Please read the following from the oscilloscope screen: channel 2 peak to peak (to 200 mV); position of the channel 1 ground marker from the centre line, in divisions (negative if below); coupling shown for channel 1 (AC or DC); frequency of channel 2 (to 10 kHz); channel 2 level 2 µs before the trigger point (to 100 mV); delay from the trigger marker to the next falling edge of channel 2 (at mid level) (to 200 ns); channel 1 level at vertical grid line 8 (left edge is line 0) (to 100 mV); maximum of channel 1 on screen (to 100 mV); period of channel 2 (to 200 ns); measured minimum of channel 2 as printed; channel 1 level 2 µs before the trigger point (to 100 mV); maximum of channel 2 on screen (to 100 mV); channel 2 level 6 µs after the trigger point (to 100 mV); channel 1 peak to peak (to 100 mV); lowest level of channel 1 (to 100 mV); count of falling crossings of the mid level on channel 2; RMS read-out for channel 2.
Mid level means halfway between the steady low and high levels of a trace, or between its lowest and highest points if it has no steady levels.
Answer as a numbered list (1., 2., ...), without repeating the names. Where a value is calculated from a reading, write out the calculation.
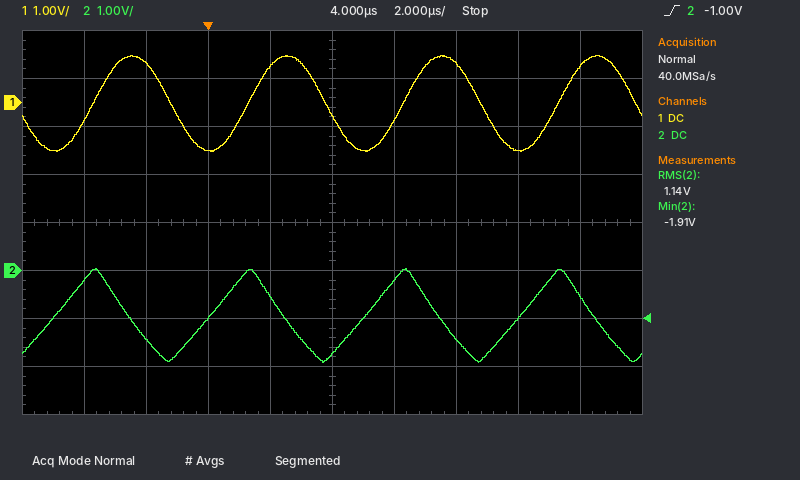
1. 2.0 V
2. +2.5 div
3. DC
4. 1 / 5.0 µs ≈ 200 kHz
5. -1.4 V
6. 2.4 µs
7. -1.0 V
8. 1.0 V
9. 5.0 µs
10. -1.91 V
11. 800 mV
12. 0.0 V
13. -200 mV
14. 1.0 V − (-1.0 V) = 2.0 V
15. -1.0 V
16. 4
17. 1.14 V
